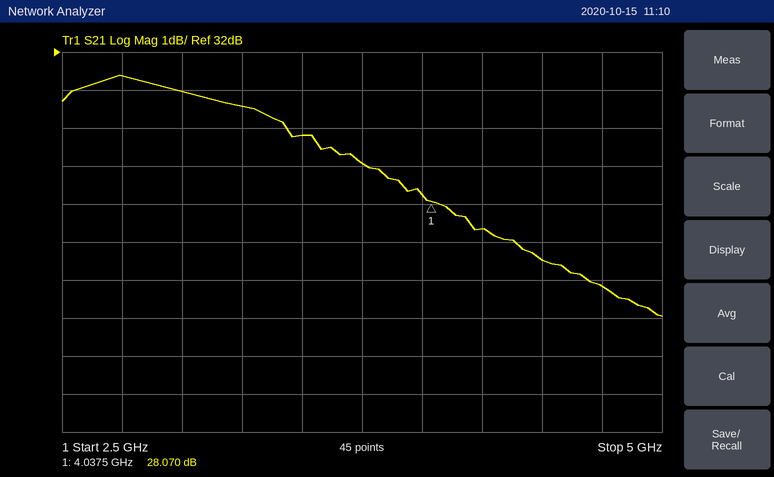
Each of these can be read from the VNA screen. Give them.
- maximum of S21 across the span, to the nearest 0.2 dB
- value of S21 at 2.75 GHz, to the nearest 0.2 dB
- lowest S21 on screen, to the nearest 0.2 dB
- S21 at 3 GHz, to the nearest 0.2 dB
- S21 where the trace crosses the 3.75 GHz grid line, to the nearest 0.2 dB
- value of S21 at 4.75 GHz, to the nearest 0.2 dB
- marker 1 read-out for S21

31.4 dB
31.4 dB
25.0 dB
31.0 dB
29.0 dB
25.8 dB
28.070 dB
